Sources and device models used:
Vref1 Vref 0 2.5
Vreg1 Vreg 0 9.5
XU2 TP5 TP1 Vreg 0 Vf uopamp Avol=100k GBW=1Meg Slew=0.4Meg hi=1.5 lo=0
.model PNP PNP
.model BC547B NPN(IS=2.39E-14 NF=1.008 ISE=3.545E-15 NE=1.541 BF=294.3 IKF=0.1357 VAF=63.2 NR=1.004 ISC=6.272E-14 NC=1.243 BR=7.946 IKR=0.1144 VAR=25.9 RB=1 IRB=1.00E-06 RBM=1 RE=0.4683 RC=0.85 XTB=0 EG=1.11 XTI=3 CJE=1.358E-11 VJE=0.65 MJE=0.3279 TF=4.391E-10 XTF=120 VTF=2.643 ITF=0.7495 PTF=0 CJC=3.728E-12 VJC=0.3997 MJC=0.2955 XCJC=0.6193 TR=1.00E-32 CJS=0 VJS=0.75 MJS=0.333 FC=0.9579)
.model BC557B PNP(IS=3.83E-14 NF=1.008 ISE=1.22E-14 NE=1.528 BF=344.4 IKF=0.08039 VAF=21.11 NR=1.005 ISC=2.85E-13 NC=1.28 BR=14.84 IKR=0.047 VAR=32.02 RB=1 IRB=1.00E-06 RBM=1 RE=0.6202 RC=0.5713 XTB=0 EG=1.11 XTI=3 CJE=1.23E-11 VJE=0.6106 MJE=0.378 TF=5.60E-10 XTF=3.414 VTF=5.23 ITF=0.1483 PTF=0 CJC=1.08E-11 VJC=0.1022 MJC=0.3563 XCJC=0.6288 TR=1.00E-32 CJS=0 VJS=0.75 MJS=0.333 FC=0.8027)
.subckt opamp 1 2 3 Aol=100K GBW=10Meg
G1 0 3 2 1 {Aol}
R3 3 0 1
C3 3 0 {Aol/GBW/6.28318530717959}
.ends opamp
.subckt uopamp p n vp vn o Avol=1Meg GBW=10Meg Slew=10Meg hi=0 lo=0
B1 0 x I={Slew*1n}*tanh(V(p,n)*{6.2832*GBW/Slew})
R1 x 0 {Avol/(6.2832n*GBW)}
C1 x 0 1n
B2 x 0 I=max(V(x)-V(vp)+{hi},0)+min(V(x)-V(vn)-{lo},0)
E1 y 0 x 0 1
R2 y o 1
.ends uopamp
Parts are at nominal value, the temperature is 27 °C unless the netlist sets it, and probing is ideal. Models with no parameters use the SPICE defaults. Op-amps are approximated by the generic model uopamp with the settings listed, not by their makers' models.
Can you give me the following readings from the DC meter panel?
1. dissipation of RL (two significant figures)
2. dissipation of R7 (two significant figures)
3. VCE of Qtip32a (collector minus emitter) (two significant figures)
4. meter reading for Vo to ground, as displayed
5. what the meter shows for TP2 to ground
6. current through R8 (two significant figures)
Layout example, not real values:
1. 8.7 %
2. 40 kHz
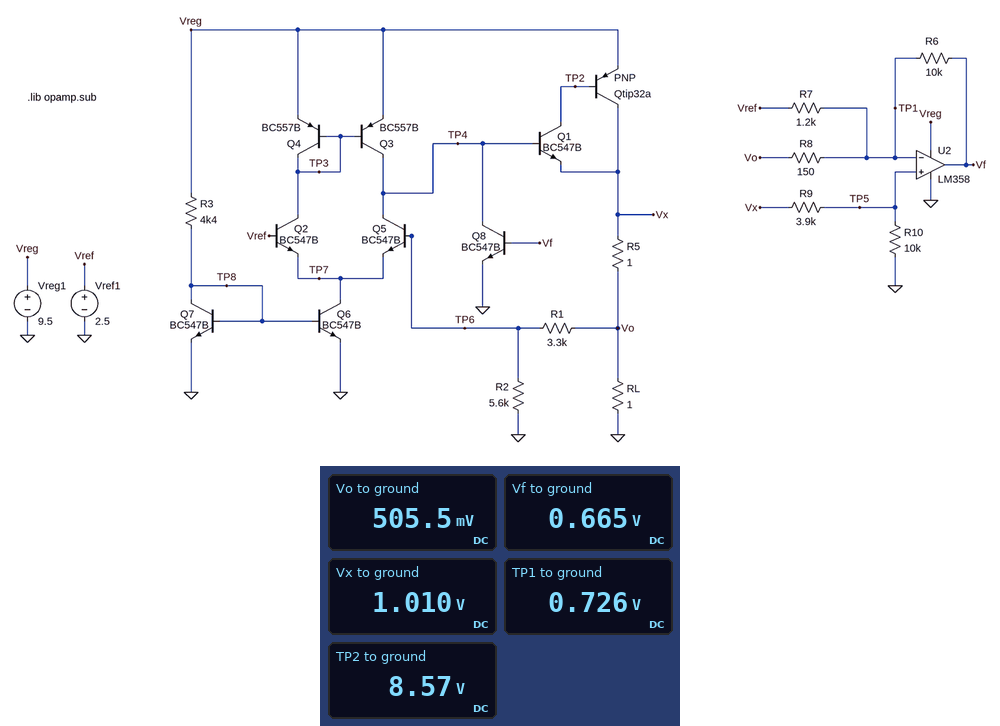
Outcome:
1. 260 mW
2. 2.6 mW
3. -8.5 V
4. 505.5 mV
5. 8.57 V
6. 1.5 mA
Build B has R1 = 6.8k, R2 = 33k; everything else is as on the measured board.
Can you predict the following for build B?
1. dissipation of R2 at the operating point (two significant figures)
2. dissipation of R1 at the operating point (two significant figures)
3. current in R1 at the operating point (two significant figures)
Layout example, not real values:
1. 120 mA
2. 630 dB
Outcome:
1. 5.3 µW
2. 1.1 µW
3. 13 µA
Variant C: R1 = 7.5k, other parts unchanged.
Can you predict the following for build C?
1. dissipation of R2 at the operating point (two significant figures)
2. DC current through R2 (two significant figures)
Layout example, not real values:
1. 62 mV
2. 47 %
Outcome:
1. 8.3 µW
2. 39 µA
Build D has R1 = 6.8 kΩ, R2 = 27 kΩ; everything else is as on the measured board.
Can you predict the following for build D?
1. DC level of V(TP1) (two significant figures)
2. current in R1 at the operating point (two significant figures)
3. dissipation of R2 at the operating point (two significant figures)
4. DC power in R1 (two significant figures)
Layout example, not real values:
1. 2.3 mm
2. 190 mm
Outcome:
1. 730 mV
2. 15 µA
3. 6.0 µW
4. 1.5 µW
